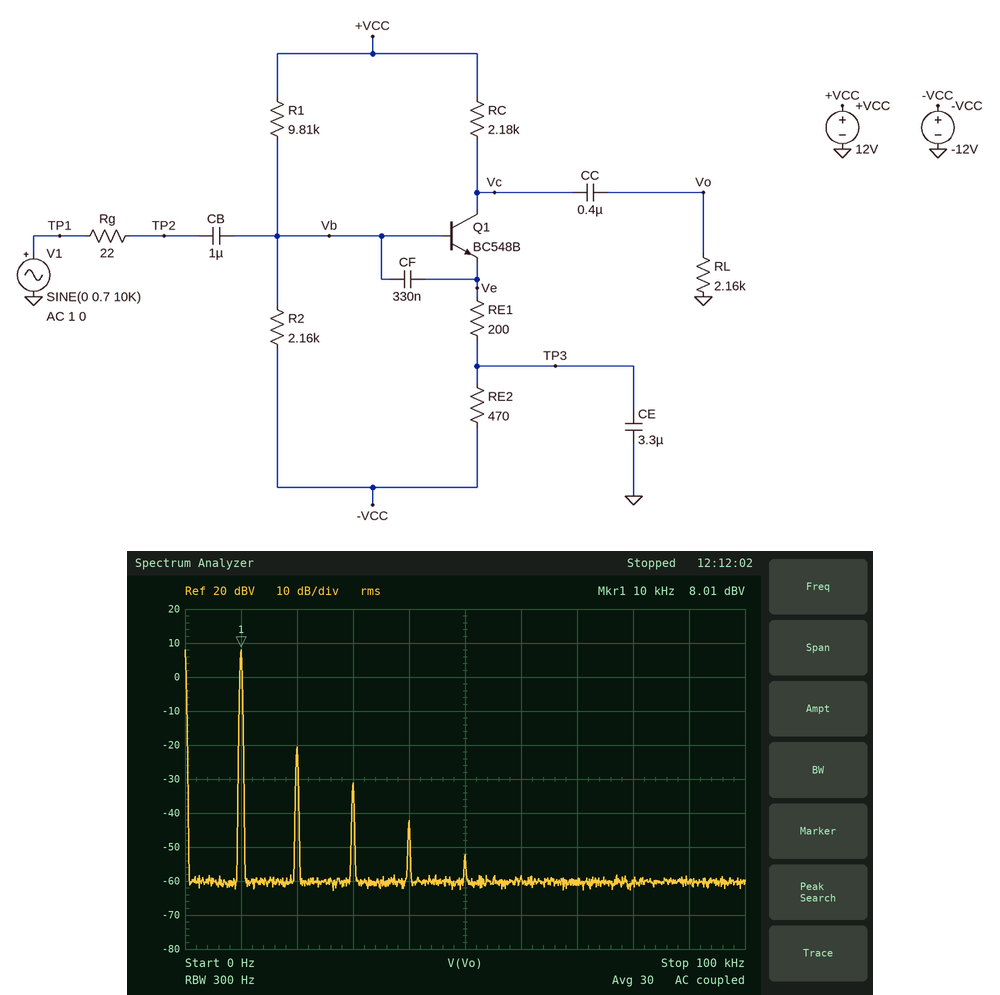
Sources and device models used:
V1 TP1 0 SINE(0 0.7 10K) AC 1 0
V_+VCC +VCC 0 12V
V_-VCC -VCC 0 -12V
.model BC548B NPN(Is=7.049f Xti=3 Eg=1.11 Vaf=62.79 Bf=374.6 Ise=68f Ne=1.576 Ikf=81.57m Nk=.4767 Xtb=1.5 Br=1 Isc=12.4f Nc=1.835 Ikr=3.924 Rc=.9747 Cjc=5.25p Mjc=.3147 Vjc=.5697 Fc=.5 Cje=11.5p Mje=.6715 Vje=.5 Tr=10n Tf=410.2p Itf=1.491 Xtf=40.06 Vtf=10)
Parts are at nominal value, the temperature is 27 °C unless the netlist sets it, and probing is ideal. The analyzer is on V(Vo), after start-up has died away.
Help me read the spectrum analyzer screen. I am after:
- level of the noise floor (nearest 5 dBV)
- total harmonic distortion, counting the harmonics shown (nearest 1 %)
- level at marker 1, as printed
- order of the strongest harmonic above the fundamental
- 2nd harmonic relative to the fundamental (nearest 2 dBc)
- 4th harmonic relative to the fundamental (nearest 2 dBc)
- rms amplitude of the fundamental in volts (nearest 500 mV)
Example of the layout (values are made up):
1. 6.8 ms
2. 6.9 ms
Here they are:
1. -60 dBV
2. 4 %
3. 8.01 dBV
4. 2
5. -28 dBc
6. -50 dBc
7. 2.5 V
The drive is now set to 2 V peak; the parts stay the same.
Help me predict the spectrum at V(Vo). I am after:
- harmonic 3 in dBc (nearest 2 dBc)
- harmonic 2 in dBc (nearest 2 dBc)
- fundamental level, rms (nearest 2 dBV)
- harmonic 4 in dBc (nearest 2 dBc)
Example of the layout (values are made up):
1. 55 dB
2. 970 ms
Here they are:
1. -18 dBc
2. -10 dBc
3. 14 dBV
4. -18 dBc
